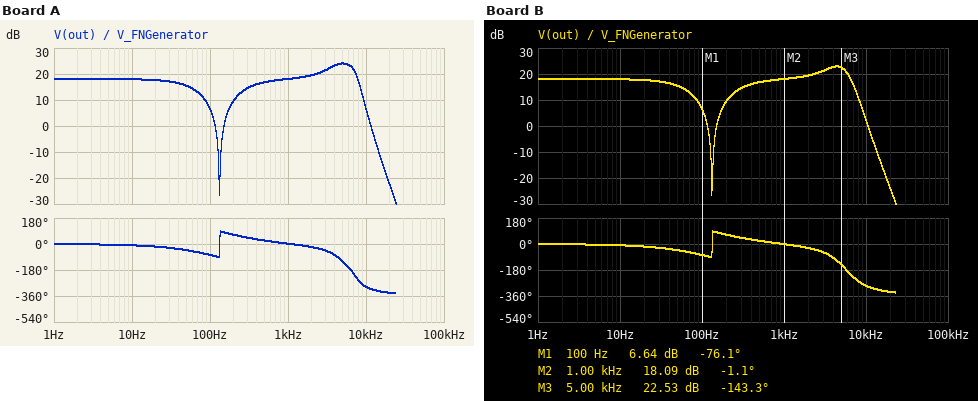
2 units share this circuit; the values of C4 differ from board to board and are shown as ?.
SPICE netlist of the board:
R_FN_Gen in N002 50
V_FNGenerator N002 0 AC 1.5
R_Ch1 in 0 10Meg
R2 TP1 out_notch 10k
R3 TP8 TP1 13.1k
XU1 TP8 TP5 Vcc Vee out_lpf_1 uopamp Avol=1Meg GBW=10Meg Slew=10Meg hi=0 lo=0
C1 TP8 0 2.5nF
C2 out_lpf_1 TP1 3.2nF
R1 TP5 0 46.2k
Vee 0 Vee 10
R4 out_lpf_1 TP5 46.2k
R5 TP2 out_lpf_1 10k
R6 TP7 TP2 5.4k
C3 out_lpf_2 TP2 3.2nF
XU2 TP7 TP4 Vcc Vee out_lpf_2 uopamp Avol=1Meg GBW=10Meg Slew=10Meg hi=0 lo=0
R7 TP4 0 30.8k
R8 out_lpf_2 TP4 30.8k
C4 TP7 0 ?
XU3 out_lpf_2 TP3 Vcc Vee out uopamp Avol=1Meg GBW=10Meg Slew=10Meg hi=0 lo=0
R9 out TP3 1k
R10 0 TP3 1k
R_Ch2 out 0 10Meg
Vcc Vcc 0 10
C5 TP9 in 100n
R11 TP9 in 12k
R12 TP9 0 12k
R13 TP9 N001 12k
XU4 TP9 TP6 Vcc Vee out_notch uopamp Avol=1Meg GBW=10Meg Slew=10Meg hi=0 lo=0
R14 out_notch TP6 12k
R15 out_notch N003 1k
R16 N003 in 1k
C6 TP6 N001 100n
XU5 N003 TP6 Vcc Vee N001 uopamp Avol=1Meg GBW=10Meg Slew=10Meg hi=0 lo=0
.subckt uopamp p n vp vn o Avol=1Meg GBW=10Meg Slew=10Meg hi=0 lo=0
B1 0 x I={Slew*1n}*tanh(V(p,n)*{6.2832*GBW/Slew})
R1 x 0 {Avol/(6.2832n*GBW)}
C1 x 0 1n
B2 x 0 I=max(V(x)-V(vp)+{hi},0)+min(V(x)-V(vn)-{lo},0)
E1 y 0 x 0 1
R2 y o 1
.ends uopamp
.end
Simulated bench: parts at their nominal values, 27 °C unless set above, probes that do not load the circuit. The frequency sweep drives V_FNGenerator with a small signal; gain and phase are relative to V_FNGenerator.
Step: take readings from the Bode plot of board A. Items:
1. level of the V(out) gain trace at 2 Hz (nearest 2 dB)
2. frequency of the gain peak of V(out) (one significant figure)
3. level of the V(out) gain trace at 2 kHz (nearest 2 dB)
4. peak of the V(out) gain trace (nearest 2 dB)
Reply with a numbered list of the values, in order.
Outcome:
1. 18 dB
2. 5 kHz
3. 20 dB
4. 24 dB
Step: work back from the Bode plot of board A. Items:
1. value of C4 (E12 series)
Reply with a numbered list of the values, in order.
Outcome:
1. 2.7 nF
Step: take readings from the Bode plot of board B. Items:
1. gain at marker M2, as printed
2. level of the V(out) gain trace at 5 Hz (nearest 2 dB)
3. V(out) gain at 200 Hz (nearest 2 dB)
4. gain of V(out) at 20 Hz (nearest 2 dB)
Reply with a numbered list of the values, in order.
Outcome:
1. 18.09 dB
2. 18 dB
3. 10 dB
4. 18 dB
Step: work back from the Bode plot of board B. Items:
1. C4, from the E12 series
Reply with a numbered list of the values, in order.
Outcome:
1. 3.3 nF
